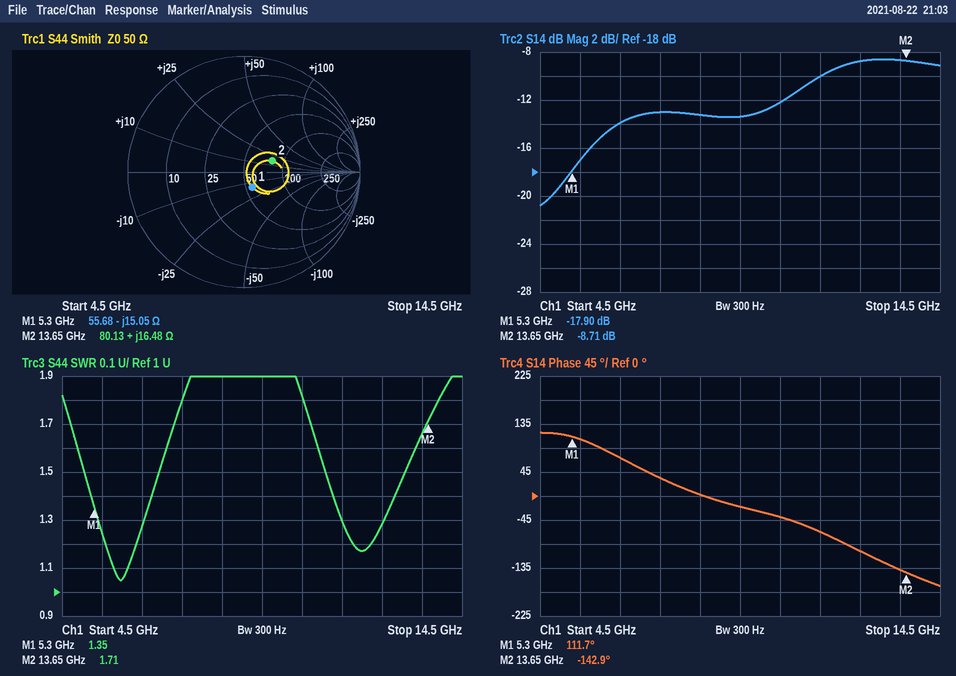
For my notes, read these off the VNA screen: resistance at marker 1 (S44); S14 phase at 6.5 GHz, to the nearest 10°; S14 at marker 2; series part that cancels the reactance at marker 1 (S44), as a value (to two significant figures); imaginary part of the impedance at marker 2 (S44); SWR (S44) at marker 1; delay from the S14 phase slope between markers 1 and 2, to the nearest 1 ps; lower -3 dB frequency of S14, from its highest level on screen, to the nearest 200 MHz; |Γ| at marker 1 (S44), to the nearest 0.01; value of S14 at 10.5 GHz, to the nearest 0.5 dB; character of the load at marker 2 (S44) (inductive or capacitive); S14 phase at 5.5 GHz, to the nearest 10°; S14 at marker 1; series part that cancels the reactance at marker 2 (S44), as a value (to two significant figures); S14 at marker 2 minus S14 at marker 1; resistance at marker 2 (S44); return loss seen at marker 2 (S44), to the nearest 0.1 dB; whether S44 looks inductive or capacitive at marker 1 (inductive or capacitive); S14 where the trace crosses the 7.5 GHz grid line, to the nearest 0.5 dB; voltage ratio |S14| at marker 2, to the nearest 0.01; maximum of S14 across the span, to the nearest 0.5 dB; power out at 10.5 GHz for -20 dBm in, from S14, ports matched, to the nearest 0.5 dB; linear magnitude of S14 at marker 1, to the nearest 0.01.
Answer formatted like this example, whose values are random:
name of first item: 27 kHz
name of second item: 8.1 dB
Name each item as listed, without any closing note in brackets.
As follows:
resistance at marker 1: 55.68 Ω
S14 phase at 6.5 GHz, to the nearest 10°: 70°
S14 at marker 2: -8.71 dB
series part that cancels the reactance at marker 1 (S44), as a value: 450 pH
imaginary part of the impedance at marker 2: +16.48 Ω
SWR (S44) at marker 1: 1.35
delay from the S14 phase slope between markers 1 and 2, to the nearest 1 ps: 85 ps
lower -3 dB frequency of S14, from its highest level on screen, to the nearest 200 MHz: 10.8 GHz
|Γ| at marker 1 (S44), to the nearest 0.01: 0.15
value of S14 at 10.5 GHz, to the nearest 0.5 dB: -12.0 dB
character of the load at marker 2 (S44): inductive
S14 phase at 5.5 GHz, to the nearest 10°: 110°
S14 at marker 1: -17.90 dB
series part that cancels the reactance at marker 2 (S44), as a value: 710 fF
S14 at marker 2 minus S14 at marker 1: 9.19 dB
resistance at marker 2: 80.13 Ω
return loss seen at marker 2 (S44), to the nearest 0.1 dB: 11.6 dB
whether S44 looks inductive or capacitive at marker 1: capacitive
S14 where the trace crosses the 7.5 GHz grid line, to the nearest 0.5 dB: -13.0 dB
voltage ratio |S14| at marker 2, to the nearest 0.01: 0.37
maximum of S14 across the span, to the nearest 0.5 dB: -8.5 dB
power out at 10.5 GHz for -20 dBm in, from S14, ports matched, to the nearest 0.5 dB: -32.0 dBm
linear magnitude of S14 at marker 1, to the nearest 0.01: 0.13
